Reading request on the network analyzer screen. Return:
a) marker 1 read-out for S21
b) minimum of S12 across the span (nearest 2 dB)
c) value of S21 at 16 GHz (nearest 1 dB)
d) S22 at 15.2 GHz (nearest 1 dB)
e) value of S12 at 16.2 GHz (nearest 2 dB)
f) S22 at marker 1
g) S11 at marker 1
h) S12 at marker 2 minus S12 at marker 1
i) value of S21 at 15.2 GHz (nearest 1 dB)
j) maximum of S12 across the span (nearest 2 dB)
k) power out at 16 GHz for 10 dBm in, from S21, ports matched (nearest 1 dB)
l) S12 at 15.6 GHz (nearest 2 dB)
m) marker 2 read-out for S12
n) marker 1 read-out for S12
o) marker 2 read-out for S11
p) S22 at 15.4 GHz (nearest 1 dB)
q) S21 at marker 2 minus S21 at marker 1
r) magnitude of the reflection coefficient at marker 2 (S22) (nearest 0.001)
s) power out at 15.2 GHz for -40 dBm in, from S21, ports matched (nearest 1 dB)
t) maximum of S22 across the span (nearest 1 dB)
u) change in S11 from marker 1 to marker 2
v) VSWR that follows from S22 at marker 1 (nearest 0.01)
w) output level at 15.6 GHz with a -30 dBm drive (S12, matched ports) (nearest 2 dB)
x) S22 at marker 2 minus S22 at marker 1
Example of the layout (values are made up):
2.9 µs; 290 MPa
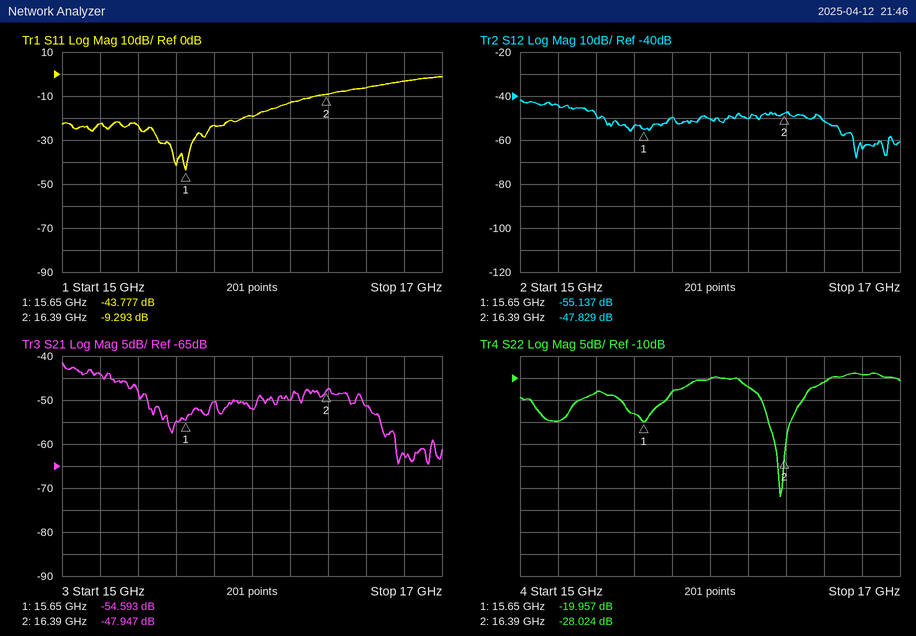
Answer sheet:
-54.593 dB; -68 dB; -52 dB; -20 dB; -50 dB; -19.957 dB; -43.777 dB; 7.308 dB; -44 dB; -42 dB; -42 dBm; -54 dB; -47.829 dB; -55.137 dB; -9.293 dB; -13 dB; 6.646 dB; 0.040; -84 dBm; -9 dB; 34.484 dB; 1.22; -84 dBm; -8.067 dB
